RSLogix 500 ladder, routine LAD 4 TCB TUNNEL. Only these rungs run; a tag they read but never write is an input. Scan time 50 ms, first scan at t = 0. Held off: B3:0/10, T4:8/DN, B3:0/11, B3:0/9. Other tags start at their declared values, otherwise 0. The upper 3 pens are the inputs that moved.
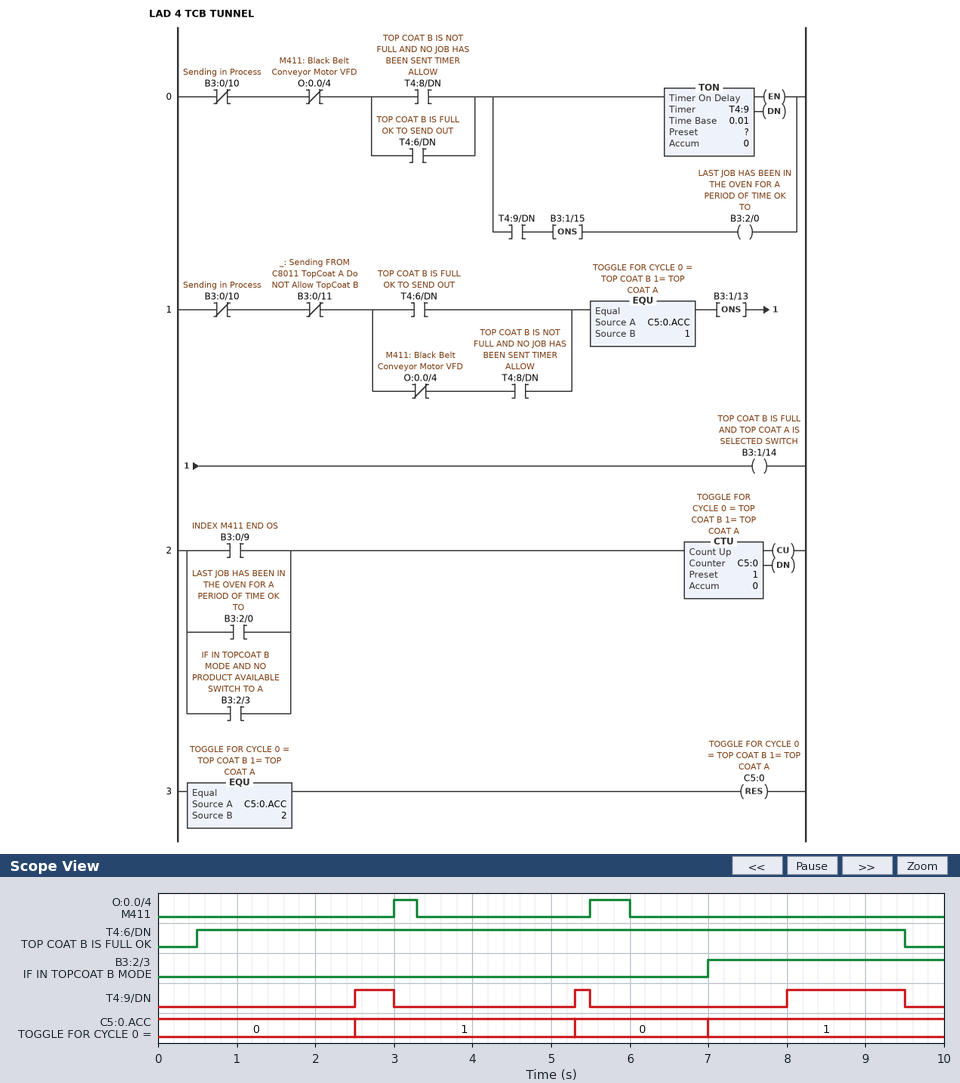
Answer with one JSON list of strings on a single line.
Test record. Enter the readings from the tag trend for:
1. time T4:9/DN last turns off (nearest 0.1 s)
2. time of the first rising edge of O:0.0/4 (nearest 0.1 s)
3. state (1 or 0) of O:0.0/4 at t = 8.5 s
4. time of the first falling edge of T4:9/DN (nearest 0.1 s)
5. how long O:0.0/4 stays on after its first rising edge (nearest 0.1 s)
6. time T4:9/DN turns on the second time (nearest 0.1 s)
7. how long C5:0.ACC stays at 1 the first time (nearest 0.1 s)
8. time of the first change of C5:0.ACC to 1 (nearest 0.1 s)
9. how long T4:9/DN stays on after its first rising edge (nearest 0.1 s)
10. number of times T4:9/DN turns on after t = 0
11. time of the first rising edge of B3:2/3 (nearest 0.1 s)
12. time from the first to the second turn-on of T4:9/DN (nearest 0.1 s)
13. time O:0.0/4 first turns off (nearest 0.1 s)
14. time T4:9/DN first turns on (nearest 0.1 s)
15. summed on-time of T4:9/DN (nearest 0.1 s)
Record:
["9.5 s", "3.0 s", "0", "3.0 s", "0.3 s", "5.3 s", "2.8 s", "2.5 s", "0.5 s", "3", "7.0 s", "2.8 s", "3.3 s", "2.5 s", "2.2 s"]
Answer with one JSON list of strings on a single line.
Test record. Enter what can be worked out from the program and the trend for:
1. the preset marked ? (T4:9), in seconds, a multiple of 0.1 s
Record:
["2.0 s"]
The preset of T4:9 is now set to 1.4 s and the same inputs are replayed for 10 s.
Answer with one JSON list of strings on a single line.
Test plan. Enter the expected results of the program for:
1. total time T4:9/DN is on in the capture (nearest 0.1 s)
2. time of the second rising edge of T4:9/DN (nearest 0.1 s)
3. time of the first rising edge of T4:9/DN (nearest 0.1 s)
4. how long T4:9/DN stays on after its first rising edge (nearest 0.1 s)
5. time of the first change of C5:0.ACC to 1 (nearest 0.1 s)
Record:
["4.0 s", "4.7 s", "1.9 s", "1.1 s", "1.9 s"]
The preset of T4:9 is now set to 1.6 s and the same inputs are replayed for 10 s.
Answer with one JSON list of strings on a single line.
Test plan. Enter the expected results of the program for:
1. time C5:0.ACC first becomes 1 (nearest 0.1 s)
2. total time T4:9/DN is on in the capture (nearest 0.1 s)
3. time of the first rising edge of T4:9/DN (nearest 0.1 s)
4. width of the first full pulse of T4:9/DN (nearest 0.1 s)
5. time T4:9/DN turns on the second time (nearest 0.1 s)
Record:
["2.1 s", "3.4 s", "2.1 s", "0.9 s", "4.9 s"]
